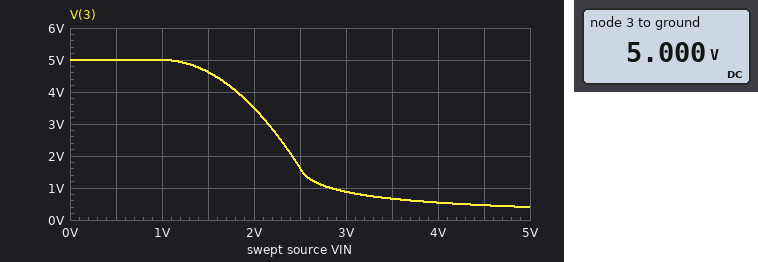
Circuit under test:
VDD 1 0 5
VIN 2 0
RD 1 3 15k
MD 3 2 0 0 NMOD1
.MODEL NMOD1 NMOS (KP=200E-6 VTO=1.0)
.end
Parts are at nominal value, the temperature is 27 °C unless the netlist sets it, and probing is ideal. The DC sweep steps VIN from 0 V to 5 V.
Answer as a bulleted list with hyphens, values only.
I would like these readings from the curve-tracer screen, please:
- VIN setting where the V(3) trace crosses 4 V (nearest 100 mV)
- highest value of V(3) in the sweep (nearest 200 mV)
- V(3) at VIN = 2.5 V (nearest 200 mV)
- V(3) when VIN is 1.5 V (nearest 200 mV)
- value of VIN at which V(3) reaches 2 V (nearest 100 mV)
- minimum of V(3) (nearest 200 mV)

- 1.8 V
- 5.0 V
- 1.6 V
- 4.6 V
- 2.4 V
- 400 mV
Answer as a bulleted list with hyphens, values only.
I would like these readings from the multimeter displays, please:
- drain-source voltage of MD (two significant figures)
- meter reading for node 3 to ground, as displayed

- 5.0 V
- 5.000 V
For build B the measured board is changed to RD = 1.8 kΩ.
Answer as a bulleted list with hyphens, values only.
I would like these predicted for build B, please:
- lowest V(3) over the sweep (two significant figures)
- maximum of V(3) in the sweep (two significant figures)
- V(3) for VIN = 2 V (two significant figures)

- 2.5 V
- 5.0 V
- 4.8 V
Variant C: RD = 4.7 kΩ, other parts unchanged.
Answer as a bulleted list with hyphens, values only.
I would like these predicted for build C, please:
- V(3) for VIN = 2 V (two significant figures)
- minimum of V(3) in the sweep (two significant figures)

- 4.5 V
- 1.2 V
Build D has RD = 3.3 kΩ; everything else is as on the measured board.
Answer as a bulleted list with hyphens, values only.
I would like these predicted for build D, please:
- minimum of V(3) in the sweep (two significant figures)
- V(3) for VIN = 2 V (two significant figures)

- 1.6 V
- 4.7 V
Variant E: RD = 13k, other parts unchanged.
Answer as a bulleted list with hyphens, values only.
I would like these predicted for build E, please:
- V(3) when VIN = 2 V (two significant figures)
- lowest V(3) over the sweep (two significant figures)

- 3.7 V
- 460 mV
